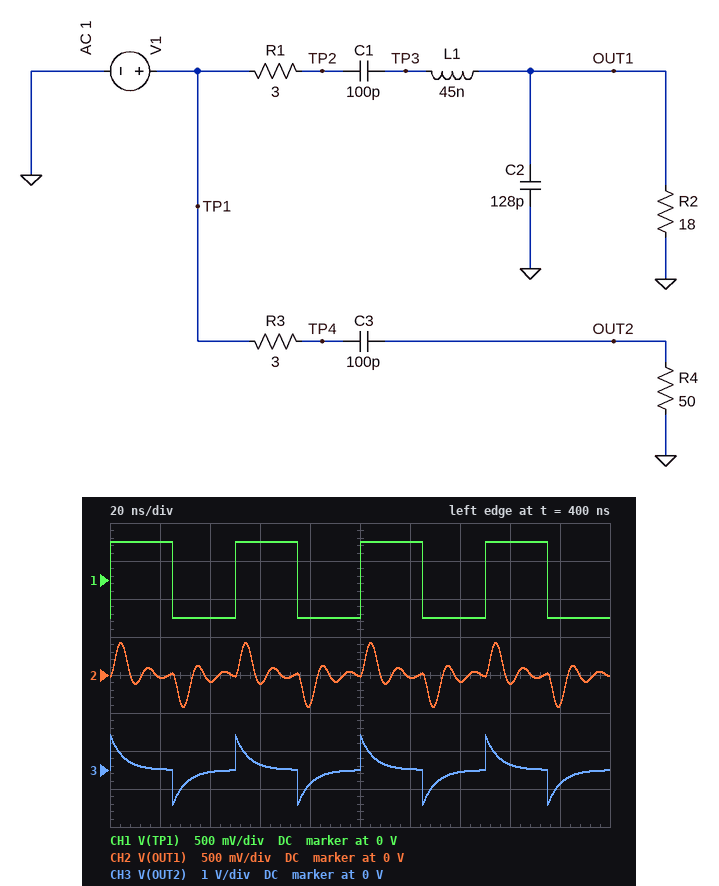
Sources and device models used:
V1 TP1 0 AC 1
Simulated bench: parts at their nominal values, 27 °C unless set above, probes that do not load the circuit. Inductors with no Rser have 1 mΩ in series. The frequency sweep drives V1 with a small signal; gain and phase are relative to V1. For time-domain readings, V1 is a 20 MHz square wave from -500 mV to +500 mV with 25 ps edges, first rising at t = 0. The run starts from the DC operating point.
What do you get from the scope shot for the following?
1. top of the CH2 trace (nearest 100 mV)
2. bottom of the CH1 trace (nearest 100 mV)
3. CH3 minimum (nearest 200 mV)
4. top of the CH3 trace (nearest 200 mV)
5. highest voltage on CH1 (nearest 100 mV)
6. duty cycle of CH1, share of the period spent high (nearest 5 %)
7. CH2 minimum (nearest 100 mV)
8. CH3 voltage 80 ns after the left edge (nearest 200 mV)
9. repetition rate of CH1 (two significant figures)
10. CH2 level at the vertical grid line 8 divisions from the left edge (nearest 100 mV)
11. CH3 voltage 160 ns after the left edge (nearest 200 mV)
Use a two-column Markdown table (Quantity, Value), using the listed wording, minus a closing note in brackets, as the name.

| Quantity | Value |
|---|---|
| top of the CH2 trace | 400 mV |
| bottom of the CH1 trace | -500 mV |
| CH3 minimum | -1.0 V |
| top of the CH3 trace | 1.0 V |
| highest voltage on CH1 | 500 mV |
| duty cycle of CH1, share of the period spent high | 50 % |
| CH2 minimum | -400 mV |
| CH3 voltage 80 ns after the left edge | -400 mV |
| repetition rate of CH1 | 20 MHz |
| CH2 level at the vertical grid line 8 divisions from the left edge | -100 mV |
| CH3 voltage 160 ns after the left edge | 200 mV |
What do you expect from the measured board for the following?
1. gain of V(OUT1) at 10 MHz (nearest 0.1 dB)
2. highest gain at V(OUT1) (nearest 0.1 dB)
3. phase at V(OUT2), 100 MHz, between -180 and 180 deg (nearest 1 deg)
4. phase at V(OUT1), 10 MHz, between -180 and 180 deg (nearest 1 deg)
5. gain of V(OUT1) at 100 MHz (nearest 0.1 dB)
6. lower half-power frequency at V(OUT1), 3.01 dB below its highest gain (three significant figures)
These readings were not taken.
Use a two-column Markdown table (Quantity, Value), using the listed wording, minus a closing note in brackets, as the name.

| Quantity | Value |
|---|---|
| gain of V(OUT1) at 10 MHz | -19.1 dB |
| highest gain at V(OUT1) | 1.1 dB |
| phase at V(OUT2), 100 MHz, between -180 and 180 deg | 17 deg |
| phase at V(OUT1), 10 MHz, between -180 and 180 deg | 74 deg |
| gain of V(OUT1) at 100 MHz | 0.5 dB |
| lower half-power frequency at V(OUT1), 3.01 dB below its highest gain | 73.0 MHz |
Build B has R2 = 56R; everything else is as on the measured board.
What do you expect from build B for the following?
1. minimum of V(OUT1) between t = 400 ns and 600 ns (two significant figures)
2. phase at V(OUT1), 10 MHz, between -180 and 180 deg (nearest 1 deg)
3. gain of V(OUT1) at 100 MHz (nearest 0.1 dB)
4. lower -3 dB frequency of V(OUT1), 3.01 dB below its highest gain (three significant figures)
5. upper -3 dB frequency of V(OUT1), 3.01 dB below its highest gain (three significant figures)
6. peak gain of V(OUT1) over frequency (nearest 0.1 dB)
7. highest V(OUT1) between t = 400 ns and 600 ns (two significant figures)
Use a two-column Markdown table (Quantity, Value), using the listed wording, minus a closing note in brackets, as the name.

| Quantity | Value |
|---|---|
| minimum of V(OUT1) between t = 400 ns and 600 ns | -670 mV |
| phase at V(OUT1), 10 MHz, between -180 and 180 deg | 50 deg |
| gain of V(OUT1) at 100 MHz | 6.6 dB |
| lower -3 dB frequency of V(OUT1), 3.01 dB below its highest gain | 88.2 MHz |
| upper -3 dB frequency of V(OUT1), 3.01 dB below its highest gain | 109 MHz |
| peak gain of V(OUT1) over frequency | 6.7 dB |
| highest V(OUT1) between t = 400 ns and 600 ns | 670 mV |
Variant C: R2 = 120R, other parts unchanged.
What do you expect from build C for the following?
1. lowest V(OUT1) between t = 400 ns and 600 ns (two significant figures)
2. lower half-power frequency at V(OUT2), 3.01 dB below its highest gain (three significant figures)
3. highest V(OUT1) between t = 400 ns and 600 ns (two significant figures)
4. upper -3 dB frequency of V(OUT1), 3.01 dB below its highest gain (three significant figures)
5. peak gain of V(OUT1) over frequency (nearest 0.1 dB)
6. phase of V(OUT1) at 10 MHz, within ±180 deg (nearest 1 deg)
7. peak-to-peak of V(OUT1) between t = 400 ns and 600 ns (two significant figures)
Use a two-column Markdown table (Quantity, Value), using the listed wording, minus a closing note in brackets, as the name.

| Quantity | Value |
|---|---|
| lowest V(OUT1) between t = 400 ns and 600 ns | -760 mV |
| lower half-power frequency at V(OUT2), 3.01 dB below its highest gain | 30.0 MHz |
| highest V(OUT1) between t = 400 ns and 600 ns | 760 mV |
| upper -3 dB frequency of V(OUT1), 3.01 dB below its highest gain | 107 MHz |
| peak gain of V(OUT1) over frequency | 9.2 dB |
| phase of V(OUT1) at 10 MHz, within ±180 deg | 29 deg |
| peak-to-peak of V(OUT1) between t = 400 ns and 600 ns | 1.5 V |
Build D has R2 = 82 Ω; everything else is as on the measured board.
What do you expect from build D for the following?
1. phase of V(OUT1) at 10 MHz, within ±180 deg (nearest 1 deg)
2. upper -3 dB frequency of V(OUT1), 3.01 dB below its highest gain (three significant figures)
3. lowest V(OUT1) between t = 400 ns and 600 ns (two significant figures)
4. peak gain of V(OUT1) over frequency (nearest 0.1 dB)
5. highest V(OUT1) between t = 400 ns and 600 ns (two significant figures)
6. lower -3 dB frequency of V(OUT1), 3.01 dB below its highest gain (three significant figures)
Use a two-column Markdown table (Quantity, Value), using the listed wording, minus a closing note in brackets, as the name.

| Quantity | Value |
|---|---|
| phase of V(OUT1) at 10 MHz, within ±180 deg | 39 deg |
| upper -3 dB frequency of V(OUT1), 3.01 dB below its highest gain | 108 MHz |
| lowest V(OUT1) between t = 400 ns and 600 ns | -720 mV |
| peak gain of V(OUT1) over frequency | 8.1 dB |
| highest V(OUT1) between t = 400 ns and 600 ns | 720 mV |
| lower -3 dB frequency of V(OUT1), 3.01 dB below its highest gain | 90.4 MHz |
